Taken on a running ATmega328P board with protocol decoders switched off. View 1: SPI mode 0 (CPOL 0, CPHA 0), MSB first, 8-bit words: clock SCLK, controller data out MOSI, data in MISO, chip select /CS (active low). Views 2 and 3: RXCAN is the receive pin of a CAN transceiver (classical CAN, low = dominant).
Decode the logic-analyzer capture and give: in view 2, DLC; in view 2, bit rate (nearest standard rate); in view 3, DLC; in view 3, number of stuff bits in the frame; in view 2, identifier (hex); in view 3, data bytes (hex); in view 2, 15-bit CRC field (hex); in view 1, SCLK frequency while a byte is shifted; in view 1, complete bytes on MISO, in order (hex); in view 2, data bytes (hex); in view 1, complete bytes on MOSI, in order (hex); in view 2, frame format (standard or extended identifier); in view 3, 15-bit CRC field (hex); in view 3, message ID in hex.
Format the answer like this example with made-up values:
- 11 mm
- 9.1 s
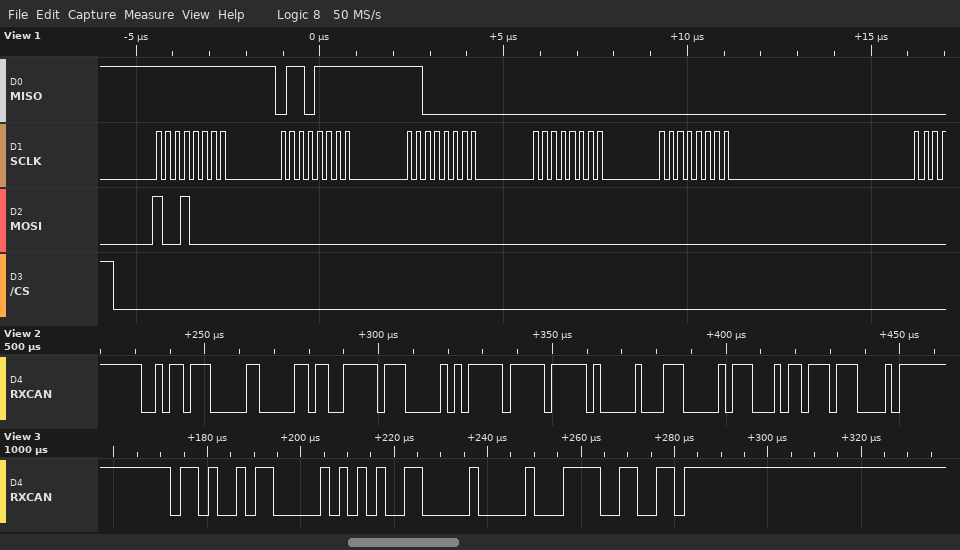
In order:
- 8
- 500 kbit/s
- 2
- 3
- 0x2DC
- A6 00
- 0x3770
- 4 MHz
- FF 6F C0 00 00
- 2C FF 02 FF FF 00 E0 71
- 90 00 00 00 00
- standard
- 0x0799
- 0x696
